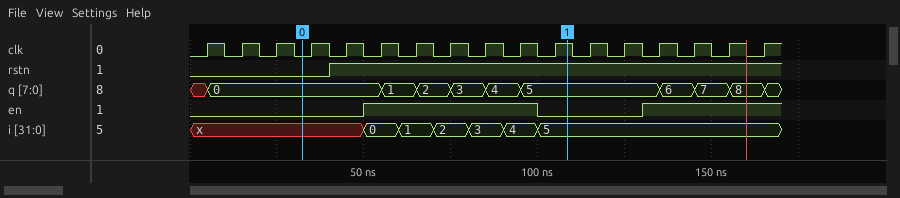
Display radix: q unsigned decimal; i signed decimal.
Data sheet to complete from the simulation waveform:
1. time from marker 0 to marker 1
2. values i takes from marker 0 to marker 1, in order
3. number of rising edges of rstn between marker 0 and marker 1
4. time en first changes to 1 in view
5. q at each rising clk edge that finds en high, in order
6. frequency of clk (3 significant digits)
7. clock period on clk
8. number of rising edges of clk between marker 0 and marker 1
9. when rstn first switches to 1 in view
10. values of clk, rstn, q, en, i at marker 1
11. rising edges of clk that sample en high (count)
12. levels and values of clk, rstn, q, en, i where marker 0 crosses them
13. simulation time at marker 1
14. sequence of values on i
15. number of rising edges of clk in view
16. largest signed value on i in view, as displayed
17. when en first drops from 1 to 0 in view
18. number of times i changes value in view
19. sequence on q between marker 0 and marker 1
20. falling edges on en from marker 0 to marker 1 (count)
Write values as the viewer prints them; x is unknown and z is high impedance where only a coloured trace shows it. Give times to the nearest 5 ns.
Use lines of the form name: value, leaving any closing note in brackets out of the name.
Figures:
time from marker 0 to marker 1: 75 ns
values i takes from marker 0 to marker 1, in order: x, 0, 1, 2, 3, 4, 5
number of rising edges of rstn between marker 0 and marker 1: 1
time en first changes to 1 in view: 50 ns
q at each rising clk edge that finds en high, in order: 0, 1, 2, 3, 4, 5, 6, 7, 8
frequency of clk: 100 MHz
clock period on clk: 10 ns
number of rising edges of clk between marker 0 and marker 1: 8
when rstn first switches to 1 in view: 40 ns
values of clk, rstn, q, en, i at marker 1: clk=1, rstn=1, q=5, en=0, i=5
rising edges of clk that sample en high: 9
levels and values of clk, rstn, q, en, i where marker 0 crosses them: clk=0, rstn=0, q=0, en=0, i=x
simulation time at marker 1: 110 ns
sequence of values on i: x, 0, 1, 2, 3, 4, 5
number of rising edges of clk in view: 17
largest signed value on i in view, as displayed: 5
when en first drops from 1 to 0 in view: 100 ns
number of times i changes value in view: 6
sequence on q between marker 0 and marker 1: 0, 1, 2, 3, 4, 5
falling edges on en from marker 0 to marker 1: 1
